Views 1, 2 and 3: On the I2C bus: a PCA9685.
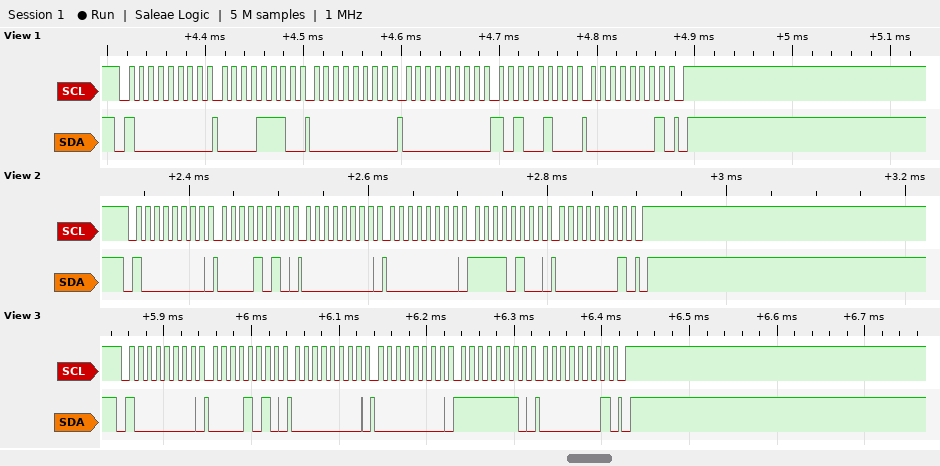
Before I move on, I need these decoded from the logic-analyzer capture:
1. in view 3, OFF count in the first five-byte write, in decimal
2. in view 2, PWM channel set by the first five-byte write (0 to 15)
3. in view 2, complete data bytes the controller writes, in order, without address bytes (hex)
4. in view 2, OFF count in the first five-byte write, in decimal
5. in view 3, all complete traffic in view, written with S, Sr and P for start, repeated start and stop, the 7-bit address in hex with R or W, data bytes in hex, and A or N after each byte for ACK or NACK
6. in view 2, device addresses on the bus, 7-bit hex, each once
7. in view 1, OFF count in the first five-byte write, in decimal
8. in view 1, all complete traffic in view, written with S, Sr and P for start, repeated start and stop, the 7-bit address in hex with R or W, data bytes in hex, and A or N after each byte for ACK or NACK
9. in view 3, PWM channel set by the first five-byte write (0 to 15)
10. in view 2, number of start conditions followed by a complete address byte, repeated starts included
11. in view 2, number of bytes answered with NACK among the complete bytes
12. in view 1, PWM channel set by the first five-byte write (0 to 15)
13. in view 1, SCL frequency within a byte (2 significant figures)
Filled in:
510
1
0A 00 00 F4 01
500
S 40W A 0A A 00 A 00 A FE A 01 A P
0x40
420
S 40W A 0E A 00 A 00 A A4 A 01 A P
1
1
0
2
100 kHz
